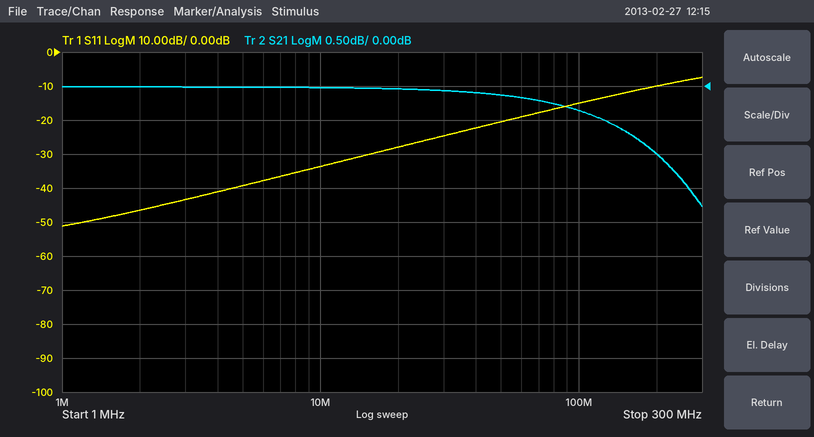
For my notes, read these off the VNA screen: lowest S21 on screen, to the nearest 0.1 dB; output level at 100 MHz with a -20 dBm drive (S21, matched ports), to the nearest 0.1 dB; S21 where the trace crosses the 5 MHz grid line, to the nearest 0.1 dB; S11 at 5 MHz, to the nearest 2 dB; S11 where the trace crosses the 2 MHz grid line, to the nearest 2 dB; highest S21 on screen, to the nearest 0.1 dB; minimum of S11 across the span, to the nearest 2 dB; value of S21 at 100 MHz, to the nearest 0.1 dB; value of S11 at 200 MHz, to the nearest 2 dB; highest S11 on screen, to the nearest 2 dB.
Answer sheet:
-1.8 dB
-20.4 dBm
0.0 dB
-40 dB
-46 dB
0.0 dB
-52 dB
-0.4 dB
-10 dB
-8 dB
